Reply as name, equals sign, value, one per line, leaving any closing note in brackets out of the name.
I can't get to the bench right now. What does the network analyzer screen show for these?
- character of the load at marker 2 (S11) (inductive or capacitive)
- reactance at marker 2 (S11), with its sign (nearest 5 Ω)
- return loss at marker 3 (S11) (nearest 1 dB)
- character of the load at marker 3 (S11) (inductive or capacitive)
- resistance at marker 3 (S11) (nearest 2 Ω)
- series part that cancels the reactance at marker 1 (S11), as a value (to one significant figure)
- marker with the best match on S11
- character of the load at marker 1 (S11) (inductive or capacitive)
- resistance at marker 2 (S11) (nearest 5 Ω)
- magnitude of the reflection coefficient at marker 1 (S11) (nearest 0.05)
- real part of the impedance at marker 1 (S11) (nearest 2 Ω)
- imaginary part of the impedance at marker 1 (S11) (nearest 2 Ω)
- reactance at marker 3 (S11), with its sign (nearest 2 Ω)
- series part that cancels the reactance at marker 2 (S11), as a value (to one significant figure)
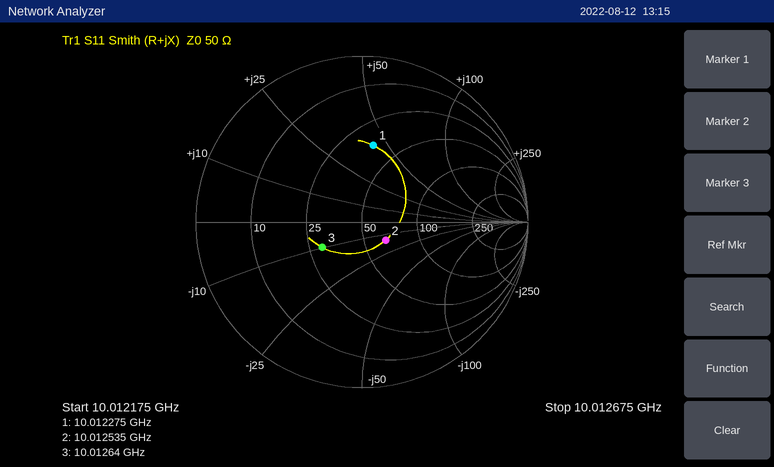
character of the load at marker 2 (S11) = capacitive
reactance at marker 2 (S11), with its sign = -15 Ω
return loss at marker 3 (S11) = 11 dB
character of the load at marker 3 (S11) = capacitive
resistance at marker 3 (S11) = 30 Ω
series part that cancels the reactance at marker 1 (S11), as a value = 400 fF
marker with the best match on S11 = marker 2
character of the load at marker 1 (S11) = inductive
resistance at marker 2 (S11) = 65 Ω
magnitude of the reflection coefficient at marker 1 (S11) = 0.45
real part of the impedance at marker 1 (S11) = 36 Ω
imaginary part of the impedance at marker 1 (S11) = +42 Ω
reactance at marker 3 (S11), with its sign = -10 Ω
series part that cancels the reactance at marker 2 (S11), as a value = 200 pH
